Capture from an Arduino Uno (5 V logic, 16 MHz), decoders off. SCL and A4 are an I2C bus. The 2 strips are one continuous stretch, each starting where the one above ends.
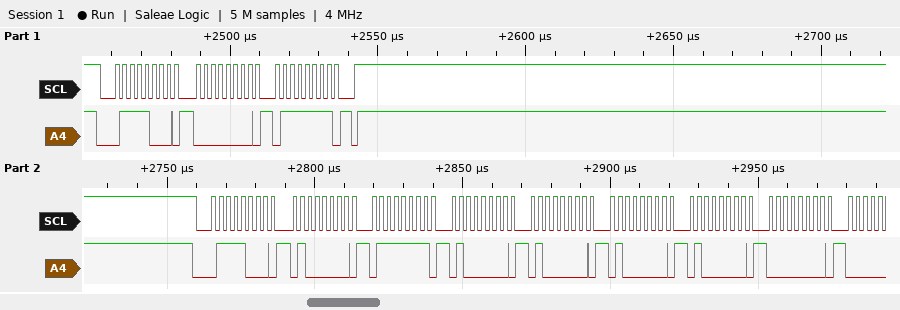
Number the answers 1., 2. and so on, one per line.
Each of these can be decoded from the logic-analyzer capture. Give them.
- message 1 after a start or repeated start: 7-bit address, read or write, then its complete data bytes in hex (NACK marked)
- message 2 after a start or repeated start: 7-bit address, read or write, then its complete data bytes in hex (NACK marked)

1. 0x3C write: 00 7F
2. 0x3C write: 40 7F 40 40 40 40 00
